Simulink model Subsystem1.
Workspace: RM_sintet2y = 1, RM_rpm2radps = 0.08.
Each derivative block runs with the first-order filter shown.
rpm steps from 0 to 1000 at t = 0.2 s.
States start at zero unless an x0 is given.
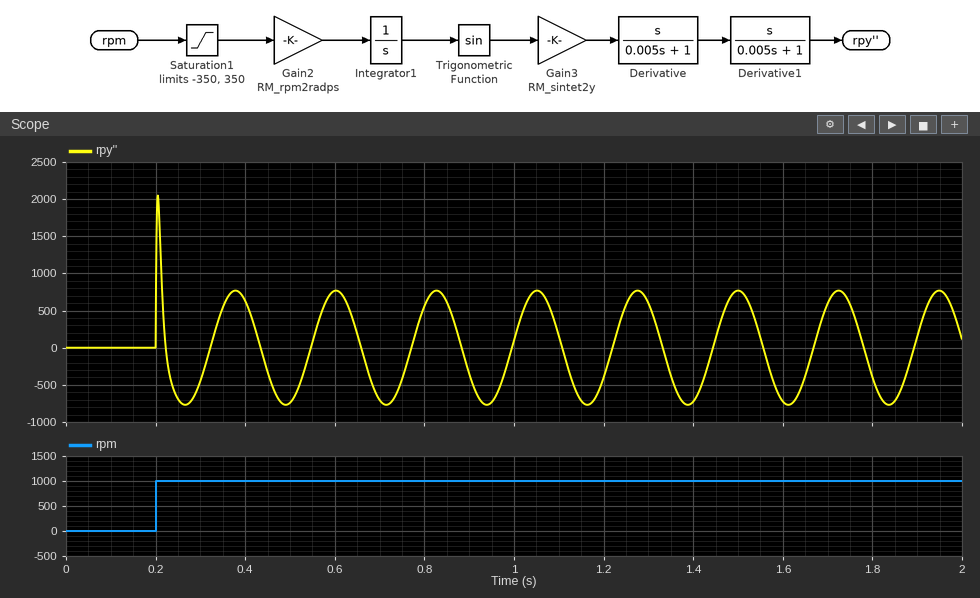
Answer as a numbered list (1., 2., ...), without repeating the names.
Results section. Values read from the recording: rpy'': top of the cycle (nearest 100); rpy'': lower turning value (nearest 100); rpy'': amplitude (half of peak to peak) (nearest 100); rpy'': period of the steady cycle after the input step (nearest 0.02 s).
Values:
1. 800
2. -800
3. 800
4. 0.22 s
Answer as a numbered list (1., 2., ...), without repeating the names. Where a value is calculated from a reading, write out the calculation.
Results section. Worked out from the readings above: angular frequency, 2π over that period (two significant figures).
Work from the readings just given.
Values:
1. 2π / 0.22 = 29 rad/s
